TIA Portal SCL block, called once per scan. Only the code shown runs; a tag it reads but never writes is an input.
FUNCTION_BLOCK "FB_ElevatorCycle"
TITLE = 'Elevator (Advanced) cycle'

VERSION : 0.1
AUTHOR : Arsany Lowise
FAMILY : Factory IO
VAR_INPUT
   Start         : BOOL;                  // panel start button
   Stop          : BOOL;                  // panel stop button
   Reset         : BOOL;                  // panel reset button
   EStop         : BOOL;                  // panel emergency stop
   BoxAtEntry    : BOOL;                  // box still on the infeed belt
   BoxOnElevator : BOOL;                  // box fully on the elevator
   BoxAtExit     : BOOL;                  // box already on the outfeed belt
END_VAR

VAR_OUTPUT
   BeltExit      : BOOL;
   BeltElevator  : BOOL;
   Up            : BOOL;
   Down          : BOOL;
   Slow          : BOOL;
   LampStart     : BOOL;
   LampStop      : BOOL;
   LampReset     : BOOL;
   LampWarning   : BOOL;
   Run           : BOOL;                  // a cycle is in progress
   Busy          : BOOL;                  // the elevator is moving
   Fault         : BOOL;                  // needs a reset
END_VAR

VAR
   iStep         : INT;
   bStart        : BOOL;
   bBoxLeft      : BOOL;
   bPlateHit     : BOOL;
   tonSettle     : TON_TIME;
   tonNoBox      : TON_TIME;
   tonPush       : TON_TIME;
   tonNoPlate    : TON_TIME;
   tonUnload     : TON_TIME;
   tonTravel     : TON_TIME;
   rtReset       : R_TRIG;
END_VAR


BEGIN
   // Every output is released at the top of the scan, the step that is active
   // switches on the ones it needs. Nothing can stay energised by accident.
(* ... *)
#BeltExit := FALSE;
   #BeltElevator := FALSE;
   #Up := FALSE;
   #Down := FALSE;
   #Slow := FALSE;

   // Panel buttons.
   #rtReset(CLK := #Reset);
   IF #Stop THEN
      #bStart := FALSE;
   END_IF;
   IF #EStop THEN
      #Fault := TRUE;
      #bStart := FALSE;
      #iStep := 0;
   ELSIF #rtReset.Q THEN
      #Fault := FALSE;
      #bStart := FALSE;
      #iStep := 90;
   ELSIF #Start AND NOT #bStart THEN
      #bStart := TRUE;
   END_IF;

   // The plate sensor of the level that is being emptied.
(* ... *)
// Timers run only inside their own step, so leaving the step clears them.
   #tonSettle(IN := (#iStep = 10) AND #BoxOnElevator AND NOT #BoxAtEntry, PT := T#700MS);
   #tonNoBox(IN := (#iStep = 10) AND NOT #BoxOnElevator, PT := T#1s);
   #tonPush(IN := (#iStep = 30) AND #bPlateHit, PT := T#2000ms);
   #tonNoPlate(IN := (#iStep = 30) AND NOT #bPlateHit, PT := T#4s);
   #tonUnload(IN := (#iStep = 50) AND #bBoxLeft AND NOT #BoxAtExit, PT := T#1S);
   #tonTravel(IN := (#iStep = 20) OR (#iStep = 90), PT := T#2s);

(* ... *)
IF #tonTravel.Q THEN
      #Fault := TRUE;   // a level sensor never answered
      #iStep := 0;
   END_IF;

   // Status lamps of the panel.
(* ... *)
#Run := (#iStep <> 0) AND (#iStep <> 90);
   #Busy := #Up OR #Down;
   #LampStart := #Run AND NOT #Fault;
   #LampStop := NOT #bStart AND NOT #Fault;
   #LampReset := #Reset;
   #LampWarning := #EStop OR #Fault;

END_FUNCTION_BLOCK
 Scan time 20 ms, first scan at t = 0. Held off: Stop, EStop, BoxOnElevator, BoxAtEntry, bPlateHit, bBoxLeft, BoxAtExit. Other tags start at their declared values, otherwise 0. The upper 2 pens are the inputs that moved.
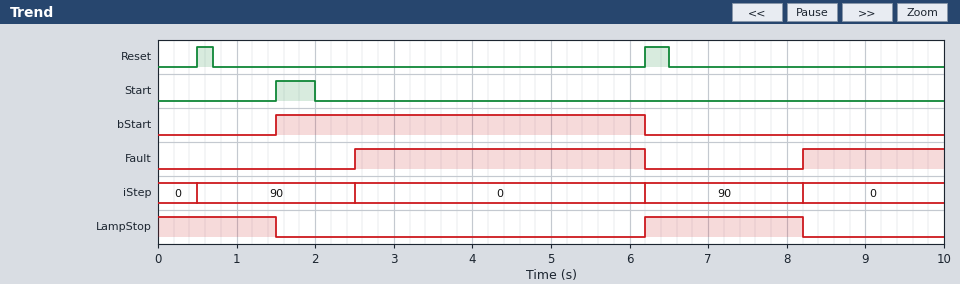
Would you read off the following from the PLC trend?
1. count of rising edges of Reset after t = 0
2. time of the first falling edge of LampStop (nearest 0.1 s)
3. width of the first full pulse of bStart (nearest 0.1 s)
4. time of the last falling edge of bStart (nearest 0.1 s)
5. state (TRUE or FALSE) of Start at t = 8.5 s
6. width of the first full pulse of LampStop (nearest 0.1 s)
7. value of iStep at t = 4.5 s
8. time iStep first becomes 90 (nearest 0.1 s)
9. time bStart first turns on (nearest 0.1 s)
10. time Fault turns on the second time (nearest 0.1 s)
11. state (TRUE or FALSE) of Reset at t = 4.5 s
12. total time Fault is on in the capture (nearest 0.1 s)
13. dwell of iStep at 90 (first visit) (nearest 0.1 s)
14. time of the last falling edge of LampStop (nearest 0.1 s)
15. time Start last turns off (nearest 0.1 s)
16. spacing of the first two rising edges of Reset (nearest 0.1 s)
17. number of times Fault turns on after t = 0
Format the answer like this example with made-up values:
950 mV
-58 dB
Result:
2
1.5 s
4.7 s
6.2 s
FALSE
2.0 s
0
0.5 s
1.5 s
8.2 s
FALSE
5.5 s
2.0 s
8.2 s
2.0 s
5.7 s
2
